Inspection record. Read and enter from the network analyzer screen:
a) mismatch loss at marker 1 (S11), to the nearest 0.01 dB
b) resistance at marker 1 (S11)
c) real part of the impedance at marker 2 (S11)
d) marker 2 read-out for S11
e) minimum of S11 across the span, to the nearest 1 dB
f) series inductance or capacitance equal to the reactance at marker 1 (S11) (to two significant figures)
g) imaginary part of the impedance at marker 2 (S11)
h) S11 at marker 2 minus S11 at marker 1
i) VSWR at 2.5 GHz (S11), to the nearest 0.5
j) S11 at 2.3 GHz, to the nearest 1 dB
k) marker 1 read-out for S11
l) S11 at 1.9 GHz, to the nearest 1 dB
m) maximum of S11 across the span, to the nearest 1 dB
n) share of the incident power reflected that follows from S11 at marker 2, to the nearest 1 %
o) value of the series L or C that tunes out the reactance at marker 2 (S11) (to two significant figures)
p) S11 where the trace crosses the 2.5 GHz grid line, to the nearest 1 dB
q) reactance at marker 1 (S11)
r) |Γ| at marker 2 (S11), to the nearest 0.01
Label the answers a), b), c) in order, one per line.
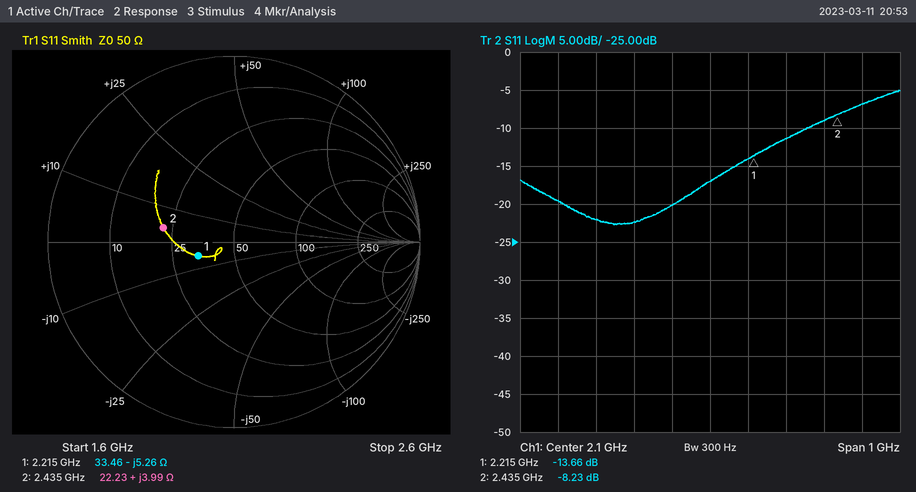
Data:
a) 0.19 dB
b) 33.46 Ω
c) 22.23 Ω
d) -8.23 dB
e) -23 dB
f) 14 pF
g) +3.99 Ω
h) 5.43 dB
i) 2.5
j) -11 dB
k) -13.66 dB
l) -22 dB
m) -5 dB
n) 15 %
o) 16 pF
p) -7 dB
q) -5.26 Ω
r) 0.39
